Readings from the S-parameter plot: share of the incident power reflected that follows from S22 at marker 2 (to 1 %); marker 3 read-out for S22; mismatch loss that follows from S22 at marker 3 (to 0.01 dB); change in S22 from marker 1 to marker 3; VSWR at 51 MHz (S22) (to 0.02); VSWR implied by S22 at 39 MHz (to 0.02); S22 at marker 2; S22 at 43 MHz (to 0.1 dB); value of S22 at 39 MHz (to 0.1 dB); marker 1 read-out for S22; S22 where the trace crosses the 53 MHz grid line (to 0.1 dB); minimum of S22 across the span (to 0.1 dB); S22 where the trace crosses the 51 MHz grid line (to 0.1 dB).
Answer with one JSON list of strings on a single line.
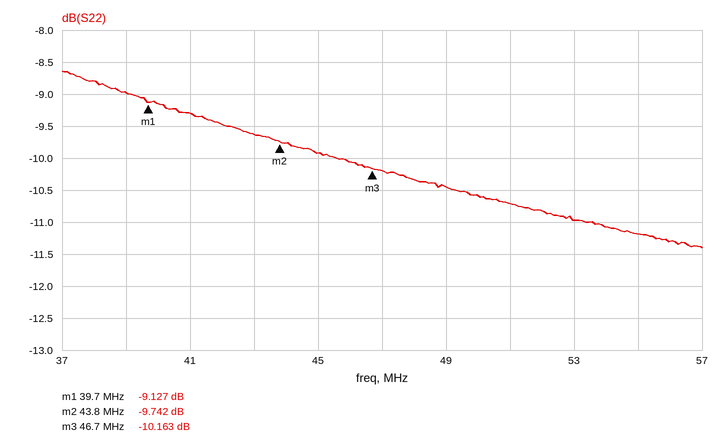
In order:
["11 %", "-10.163 dB", "0.44 dB", "-1.036 dB", "1.82", "2.10", "-9.742 dB", "-9.6 dB", "-9.0 dB", "-9.127 dB", "-11.0 dB", "-11.4 dB", "-10.7 dB"]
